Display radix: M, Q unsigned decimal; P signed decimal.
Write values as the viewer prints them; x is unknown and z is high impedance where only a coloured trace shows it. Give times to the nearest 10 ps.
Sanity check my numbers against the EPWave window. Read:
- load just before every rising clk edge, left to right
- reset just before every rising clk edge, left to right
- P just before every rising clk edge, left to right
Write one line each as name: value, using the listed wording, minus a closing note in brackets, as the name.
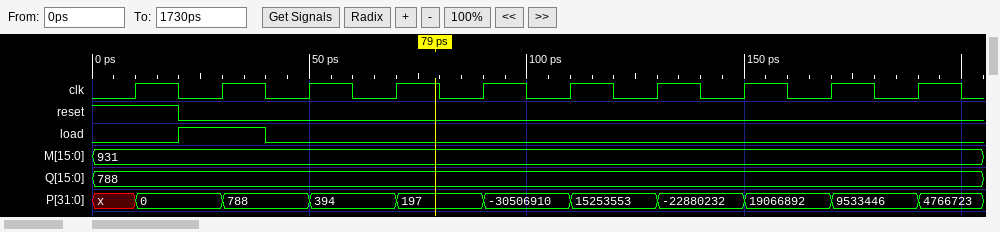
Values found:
load just before every rising clk edge, left to right: 0 1 0 0 0 0 0 0 0 0
reset just before every rising clk edge, left to right: 1 0 0 0 0 0 0 0 0 0
P just before every rising clk edge, left to right: x, 0, 788, 394, 197, -30506910, 15253553, -22880232, 19066892, 9533446
